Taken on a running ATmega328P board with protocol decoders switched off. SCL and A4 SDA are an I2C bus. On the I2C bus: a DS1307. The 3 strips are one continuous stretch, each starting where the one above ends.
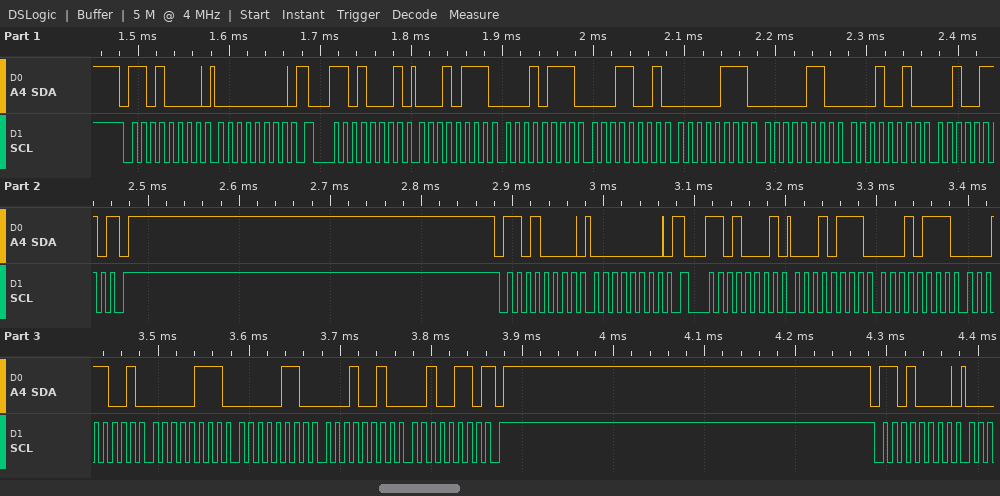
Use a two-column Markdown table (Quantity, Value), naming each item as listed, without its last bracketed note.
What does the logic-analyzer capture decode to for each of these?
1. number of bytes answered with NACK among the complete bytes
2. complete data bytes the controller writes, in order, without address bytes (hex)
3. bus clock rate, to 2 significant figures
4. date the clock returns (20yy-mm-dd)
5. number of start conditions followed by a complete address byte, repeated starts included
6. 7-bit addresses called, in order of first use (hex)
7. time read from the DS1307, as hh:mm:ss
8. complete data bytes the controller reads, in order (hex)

| Quantity | Value |
|---|---|
| number of bytes answered with NACK among the complete bytes | 2 |
| complete data bytes the controller writes, in order, without address bytes | 00 00 |
| bus clock rate, to 2 significant figures | 100 kHz |
| date the clock returns | 2026-12-06 |
| number of start conditions followed by a complete address byte, repeated starts included | 5 |
| 7-bit addresses called, in order of first use | 0x68 |
| time read from the DS1307, as hh:mm:ss | 19:17:17 |
| complete data bytes the controller reads, in order | 17 17 19 07 06 12 26 17 17 19 07 06 12 26 |
